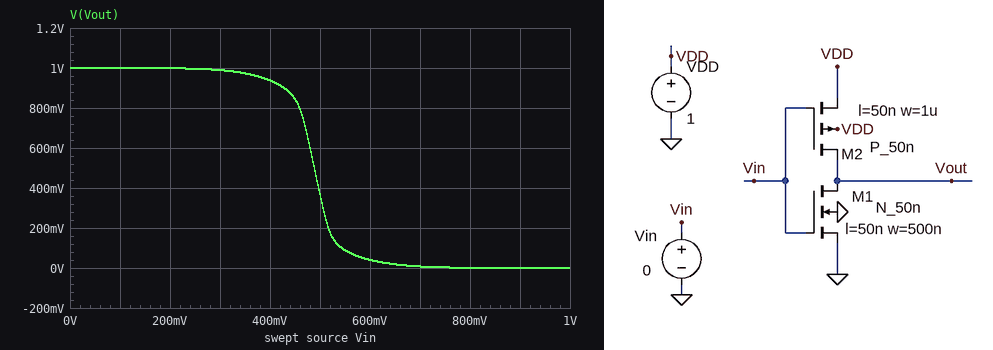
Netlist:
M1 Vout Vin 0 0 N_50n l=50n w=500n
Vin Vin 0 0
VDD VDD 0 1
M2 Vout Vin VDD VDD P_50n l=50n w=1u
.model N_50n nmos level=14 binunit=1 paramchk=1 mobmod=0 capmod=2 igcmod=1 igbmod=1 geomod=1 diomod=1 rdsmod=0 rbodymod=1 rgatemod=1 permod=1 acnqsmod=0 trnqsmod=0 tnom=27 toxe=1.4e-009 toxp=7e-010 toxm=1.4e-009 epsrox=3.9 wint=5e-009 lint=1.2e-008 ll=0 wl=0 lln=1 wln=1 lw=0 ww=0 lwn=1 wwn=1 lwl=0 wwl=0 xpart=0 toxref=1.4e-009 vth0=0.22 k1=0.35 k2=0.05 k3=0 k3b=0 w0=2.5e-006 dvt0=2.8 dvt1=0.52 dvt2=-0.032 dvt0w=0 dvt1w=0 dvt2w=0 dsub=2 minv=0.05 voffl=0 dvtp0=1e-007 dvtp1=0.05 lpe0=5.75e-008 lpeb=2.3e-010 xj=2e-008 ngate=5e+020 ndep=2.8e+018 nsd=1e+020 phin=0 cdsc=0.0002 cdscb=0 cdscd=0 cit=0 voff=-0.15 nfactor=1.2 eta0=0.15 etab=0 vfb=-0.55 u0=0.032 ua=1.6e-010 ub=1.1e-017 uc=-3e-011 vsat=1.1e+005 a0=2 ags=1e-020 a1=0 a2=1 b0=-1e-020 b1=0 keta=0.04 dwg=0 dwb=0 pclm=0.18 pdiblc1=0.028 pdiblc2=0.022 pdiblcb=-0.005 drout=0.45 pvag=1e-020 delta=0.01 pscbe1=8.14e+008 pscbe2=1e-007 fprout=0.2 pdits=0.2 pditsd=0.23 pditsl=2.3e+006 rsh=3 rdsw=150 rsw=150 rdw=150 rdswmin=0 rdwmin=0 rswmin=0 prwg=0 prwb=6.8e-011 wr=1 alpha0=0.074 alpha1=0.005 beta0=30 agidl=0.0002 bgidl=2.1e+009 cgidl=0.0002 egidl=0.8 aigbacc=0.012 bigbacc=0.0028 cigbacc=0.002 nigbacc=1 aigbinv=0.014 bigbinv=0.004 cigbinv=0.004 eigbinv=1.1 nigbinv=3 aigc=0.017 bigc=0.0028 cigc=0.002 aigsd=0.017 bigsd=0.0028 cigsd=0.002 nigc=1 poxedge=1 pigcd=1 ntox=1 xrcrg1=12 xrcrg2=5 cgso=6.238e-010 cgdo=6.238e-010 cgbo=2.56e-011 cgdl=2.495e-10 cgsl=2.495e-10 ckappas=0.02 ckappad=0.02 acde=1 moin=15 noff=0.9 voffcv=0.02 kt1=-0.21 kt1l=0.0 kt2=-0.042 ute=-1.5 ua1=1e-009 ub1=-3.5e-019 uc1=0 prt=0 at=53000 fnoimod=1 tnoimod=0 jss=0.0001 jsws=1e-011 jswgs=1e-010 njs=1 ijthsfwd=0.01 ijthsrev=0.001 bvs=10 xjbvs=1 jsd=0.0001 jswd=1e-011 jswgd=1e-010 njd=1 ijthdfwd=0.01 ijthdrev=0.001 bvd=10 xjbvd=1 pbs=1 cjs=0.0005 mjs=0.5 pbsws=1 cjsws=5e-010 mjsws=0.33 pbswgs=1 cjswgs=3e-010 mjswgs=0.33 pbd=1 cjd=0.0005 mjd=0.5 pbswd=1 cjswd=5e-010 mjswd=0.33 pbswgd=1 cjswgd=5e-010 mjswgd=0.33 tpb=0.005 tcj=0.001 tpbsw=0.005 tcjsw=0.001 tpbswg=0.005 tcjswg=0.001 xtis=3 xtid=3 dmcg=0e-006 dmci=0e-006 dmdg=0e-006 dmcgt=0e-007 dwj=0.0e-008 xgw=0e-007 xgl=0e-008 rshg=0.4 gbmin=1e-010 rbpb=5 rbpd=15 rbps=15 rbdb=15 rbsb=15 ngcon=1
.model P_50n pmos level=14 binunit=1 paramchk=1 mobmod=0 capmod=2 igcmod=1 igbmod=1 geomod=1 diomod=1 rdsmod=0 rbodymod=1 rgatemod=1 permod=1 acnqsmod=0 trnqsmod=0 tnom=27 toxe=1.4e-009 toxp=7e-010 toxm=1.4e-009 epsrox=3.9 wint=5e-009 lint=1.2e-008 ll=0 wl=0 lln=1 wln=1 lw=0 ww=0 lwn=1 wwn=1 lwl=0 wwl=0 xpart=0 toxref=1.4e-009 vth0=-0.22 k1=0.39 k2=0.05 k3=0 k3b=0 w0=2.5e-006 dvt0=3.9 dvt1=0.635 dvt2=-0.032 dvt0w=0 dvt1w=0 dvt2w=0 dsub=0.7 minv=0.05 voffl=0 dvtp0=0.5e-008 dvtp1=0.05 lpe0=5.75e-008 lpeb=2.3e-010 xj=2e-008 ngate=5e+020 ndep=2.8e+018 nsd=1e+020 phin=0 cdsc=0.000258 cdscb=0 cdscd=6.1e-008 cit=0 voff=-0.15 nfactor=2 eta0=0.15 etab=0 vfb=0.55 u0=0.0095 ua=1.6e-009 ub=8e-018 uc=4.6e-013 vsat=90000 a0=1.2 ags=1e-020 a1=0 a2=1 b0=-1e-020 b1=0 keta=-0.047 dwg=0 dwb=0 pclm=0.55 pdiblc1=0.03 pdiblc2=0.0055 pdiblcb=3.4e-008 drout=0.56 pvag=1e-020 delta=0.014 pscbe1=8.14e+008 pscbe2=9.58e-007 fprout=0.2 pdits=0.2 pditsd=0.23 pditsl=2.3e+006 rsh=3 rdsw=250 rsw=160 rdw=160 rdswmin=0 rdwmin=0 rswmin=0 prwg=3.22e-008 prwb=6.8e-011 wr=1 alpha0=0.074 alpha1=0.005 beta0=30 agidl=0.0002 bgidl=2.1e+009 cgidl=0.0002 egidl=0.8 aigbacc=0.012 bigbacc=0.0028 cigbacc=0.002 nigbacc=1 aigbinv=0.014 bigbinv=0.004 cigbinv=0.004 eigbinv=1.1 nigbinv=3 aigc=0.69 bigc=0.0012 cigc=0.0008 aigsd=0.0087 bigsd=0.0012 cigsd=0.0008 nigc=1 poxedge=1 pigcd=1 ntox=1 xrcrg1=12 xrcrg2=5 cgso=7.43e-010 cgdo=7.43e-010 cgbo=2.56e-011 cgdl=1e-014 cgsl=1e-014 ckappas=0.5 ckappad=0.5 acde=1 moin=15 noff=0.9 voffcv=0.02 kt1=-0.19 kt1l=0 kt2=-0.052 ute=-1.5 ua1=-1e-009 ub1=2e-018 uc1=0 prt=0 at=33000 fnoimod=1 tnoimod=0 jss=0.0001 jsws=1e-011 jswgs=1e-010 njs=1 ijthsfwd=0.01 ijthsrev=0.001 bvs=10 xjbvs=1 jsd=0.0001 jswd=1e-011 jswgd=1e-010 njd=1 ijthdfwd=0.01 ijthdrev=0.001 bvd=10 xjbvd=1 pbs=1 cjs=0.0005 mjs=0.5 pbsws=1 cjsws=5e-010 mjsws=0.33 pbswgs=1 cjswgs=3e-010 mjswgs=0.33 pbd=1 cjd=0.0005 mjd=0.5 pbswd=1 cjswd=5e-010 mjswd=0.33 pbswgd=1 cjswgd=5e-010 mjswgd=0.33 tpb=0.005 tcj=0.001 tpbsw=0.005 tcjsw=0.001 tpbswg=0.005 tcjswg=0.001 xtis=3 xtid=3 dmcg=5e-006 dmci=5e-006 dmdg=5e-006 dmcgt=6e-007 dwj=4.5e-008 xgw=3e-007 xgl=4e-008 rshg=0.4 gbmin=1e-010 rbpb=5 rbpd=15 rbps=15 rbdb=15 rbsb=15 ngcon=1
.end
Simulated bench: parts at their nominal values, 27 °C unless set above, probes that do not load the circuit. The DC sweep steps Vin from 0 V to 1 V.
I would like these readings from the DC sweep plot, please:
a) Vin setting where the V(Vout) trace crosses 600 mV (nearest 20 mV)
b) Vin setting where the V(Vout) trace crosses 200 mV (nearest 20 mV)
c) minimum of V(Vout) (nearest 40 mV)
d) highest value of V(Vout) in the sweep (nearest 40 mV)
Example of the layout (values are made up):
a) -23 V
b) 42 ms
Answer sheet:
a) 480 mV
b) 520 mV
c) 0 V
d) 1.00 V
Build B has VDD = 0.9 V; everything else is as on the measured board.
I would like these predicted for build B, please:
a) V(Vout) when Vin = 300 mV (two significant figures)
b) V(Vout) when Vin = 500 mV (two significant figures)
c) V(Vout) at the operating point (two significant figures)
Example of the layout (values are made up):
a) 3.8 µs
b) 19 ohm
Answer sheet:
a) 890 mV
b) 56 mV
c) 900 mV
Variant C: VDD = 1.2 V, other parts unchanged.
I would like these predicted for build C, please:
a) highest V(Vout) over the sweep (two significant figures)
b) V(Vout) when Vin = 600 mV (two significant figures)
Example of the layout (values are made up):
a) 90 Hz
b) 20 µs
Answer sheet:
a) 1.2 V
b) 470 mV
